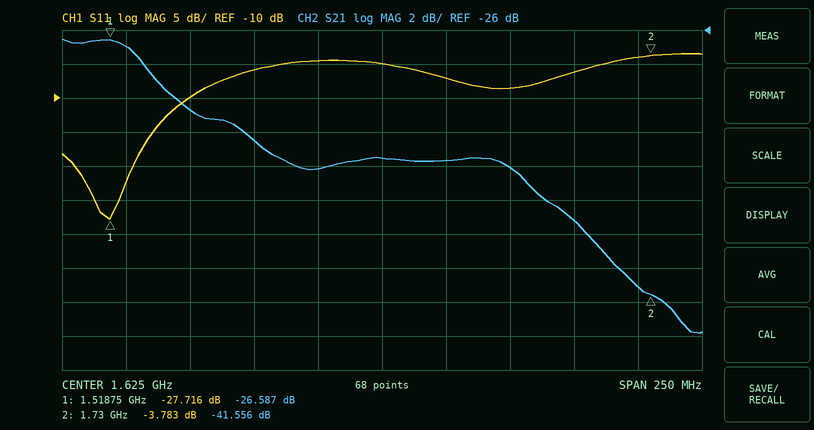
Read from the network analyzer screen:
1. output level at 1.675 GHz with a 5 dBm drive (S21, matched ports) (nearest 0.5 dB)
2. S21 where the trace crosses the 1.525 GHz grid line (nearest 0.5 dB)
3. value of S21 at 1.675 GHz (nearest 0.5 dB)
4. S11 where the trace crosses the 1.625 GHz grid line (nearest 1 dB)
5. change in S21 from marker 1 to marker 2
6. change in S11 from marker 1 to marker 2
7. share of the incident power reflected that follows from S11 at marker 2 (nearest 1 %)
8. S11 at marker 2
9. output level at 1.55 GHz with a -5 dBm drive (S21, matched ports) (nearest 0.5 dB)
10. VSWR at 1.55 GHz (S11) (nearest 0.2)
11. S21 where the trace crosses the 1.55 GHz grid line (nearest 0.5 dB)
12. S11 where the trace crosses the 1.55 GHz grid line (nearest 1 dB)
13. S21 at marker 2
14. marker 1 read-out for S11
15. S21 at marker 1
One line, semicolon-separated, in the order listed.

-29.0 dBm; -27.0 dB; -34.0 dB; -5 dB; -14.969 dB; 23.933 dB; 42 %; -3.783 dB; -35.5 dBm; 2.0; -30.5 dB; -10 dB; -41.556 dB; -27.716 dB; -26.587 dB
